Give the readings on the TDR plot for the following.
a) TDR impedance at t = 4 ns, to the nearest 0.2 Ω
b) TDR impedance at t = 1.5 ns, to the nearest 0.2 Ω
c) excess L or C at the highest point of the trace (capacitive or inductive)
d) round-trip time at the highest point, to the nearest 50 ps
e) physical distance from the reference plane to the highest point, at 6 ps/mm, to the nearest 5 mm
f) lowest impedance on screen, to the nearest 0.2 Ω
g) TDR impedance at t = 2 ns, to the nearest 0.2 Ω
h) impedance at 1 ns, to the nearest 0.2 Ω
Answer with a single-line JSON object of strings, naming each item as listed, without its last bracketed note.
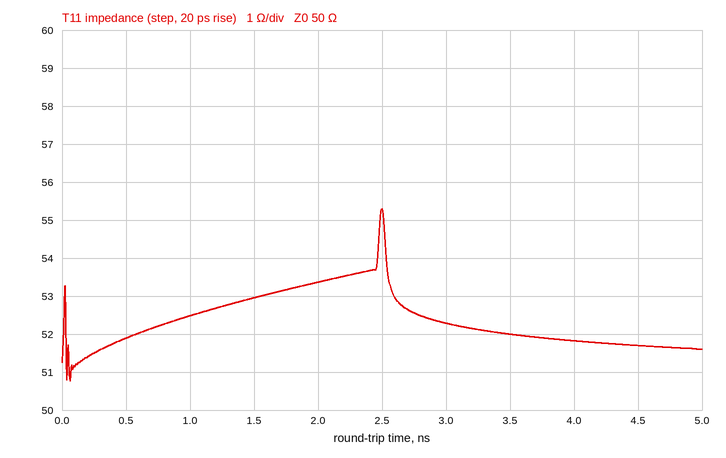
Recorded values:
{"TDR impedance at t = 4 ns, to the nearest 0.2 Ω": "51.8 Ω", "TDR impedance at t = 1.5 ns, to the nearest 0.2 Ω": "53.0 Ω", "excess L or C at the highest point of the trace": "inductive", "round-trip time at the highest point, to the nearest 50 ps": "2.50 ns", "physical distance from the reference plane to the highest point, at 6 ps/mm, to the nearest 5 mm": "210 mm", "lowest impedance on screen, to the nearest 0.2 Ω": "50.8 Ω", "TDR impedance at t = 2 ns, to the nearest 0.2 Ω": "53.4 Ω", "impedance at 1 ns, to the nearest 0.2 Ω": "52.4 Ω"}
